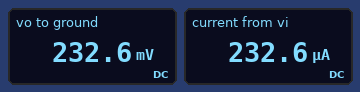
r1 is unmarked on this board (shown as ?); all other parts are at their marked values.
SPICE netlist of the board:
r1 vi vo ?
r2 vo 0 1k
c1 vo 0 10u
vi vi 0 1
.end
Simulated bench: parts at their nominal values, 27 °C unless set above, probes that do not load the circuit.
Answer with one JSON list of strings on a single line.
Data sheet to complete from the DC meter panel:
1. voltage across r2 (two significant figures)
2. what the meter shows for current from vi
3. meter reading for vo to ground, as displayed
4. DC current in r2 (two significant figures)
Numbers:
["230 mV", "232.6 µA", "232.6 mV", "230 µA"]
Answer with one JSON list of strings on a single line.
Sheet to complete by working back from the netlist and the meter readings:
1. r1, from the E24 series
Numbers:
["3.3 kΩ"]
